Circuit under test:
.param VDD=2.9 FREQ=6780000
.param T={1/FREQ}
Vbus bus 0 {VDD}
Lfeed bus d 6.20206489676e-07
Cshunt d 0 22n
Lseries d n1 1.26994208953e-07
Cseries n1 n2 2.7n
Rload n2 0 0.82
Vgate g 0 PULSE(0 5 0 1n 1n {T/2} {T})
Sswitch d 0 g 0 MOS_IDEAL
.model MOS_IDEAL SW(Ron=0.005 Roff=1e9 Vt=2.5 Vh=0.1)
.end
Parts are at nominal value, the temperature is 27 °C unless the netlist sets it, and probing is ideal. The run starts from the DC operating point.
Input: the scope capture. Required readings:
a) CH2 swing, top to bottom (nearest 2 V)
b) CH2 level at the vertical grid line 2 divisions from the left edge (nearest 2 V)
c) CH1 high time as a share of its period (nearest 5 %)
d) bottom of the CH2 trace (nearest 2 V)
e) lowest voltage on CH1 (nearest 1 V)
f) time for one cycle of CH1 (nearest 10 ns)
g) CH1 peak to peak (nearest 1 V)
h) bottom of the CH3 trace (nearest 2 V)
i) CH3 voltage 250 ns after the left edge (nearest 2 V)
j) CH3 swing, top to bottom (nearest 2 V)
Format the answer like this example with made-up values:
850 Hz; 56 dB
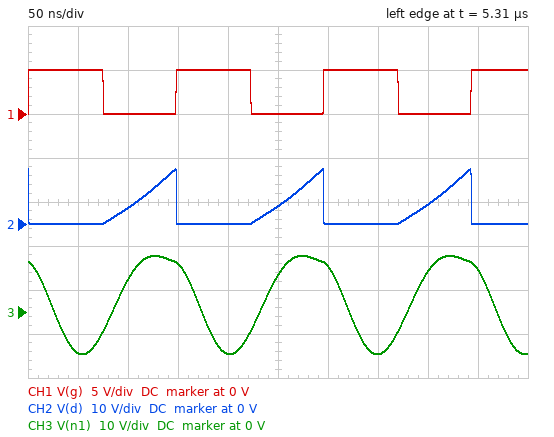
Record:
12 V; 4 V; 50 %; 0 V; 0 V; 150 ns; 5 V; -10 V; 8 V; 22 V
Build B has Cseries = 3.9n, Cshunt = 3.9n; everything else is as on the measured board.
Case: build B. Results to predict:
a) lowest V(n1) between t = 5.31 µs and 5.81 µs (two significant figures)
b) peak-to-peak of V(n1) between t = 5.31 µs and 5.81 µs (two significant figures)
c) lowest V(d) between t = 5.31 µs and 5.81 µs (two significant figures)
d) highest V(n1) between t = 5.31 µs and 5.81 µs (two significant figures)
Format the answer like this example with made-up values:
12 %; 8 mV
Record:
-19 V; 42 V; 12 mV; 23 V
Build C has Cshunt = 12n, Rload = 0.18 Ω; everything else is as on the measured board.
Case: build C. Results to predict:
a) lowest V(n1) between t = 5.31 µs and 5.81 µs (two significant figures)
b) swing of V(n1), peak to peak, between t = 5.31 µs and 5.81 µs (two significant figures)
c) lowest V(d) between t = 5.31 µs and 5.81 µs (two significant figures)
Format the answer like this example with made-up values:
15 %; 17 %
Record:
-10 V; 24 V; 8.0 mV
